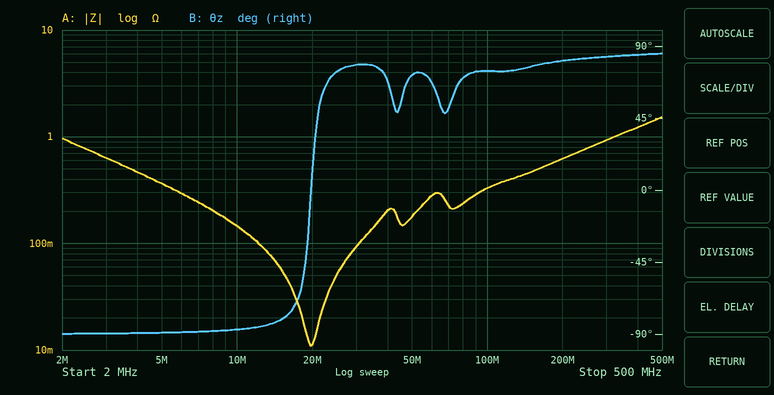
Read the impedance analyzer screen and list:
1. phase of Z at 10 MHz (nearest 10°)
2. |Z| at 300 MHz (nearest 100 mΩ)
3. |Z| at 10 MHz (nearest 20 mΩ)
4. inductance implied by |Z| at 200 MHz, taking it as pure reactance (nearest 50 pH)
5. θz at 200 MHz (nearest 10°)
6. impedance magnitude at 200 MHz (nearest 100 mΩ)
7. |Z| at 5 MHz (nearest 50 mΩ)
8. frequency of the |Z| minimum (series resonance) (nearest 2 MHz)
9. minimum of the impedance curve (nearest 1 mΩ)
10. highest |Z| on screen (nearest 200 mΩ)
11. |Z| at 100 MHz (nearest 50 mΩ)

-90°
900 mΩ
140 mΩ
500 pH
80°
600 mΩ
350 mΩ
20 MHz
11 mΩ
1.6 Ω
350 mΩ
